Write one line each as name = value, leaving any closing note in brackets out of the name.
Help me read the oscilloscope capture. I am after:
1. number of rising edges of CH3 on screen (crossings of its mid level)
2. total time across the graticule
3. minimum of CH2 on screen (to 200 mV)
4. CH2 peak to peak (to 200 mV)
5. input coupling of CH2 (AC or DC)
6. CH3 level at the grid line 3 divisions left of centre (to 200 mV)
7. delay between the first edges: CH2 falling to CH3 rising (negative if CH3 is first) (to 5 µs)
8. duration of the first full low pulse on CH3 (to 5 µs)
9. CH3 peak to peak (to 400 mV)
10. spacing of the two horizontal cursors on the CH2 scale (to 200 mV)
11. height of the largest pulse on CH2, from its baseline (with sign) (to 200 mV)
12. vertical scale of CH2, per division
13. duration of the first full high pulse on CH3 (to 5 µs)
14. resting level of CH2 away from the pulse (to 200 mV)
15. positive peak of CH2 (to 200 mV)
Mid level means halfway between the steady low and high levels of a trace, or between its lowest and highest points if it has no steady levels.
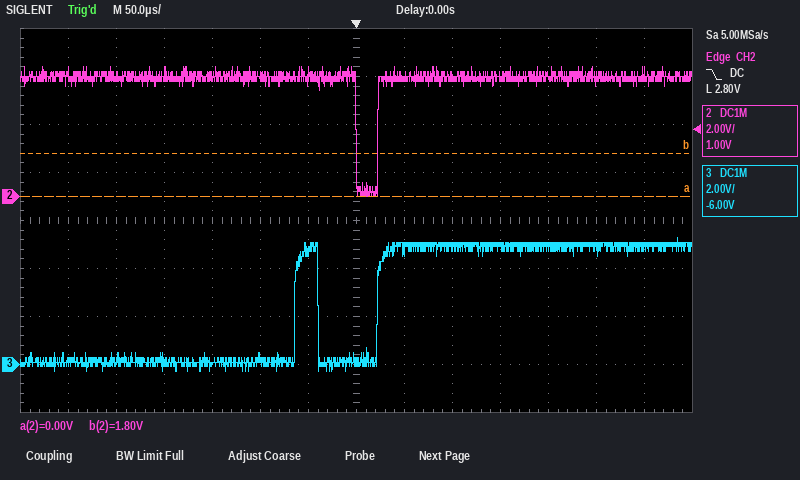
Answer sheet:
number of rising edges of CH3 on screen = 2
total time across the graticule = 700 µs
minimum of CH2 on screen = 0.0 V
CH2 peak to peak = 5.4 V
input coupling of CH2 = DC
CH3 level at the grid line 3 divisions left of centre = 0.0 V
delay between the first edges: CH2 falling to CH3 rising (negative if CH3 is first) = -65 µs
duration of the first full low pulse on CH3 = 60 µs
CH3 peak to peak = 5.6 V
spacing of the two horizontal cursors on the CH2 scale = 1.8 V
height of the largest pulse on CH2, from its baseline (with sign) = -5.0 V
vertical scale of CH2, per division = 2 V
duration of the first full high pulse on CH3 = 25 µs
resting level of CH2 away from the pulse = 5.0 V
positive peak of CH2 = 5.4 V
